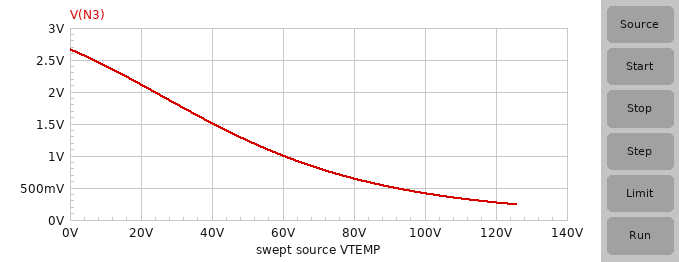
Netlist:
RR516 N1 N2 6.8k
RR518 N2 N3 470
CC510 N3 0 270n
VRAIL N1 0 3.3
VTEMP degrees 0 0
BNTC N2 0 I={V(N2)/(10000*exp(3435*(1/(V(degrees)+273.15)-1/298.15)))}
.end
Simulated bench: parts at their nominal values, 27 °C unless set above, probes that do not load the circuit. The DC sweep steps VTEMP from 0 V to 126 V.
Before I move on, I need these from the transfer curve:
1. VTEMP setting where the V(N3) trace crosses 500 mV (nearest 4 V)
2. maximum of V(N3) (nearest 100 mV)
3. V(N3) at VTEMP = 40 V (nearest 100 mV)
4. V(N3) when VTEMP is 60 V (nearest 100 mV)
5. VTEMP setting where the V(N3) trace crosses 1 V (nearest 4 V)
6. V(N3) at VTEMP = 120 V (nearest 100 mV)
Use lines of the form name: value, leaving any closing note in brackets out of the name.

VTEMP setting where the V(N3) trace crosses 500 mV: 92 V
maximum of V(N3): 2.7 V
V(N3) at VTEMP = 40 V: 1.5 V
V(N3) when VTEMP is 60 V: 1.0 V
VTEMP setting where the V(N3) trace crosses 1 V: 60 V
V(N3) at VTEMP = 120 V: 300 mV
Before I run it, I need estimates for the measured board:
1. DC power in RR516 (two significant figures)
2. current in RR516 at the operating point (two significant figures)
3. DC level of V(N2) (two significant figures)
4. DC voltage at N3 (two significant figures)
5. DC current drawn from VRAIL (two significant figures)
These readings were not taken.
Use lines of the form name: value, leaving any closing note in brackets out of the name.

DC power in RR516: 59 µW
current in RR516 at the operating point: 93 µA
DC level of V(N2): 2.7 V
DC voltage at N3: 2.7 V
DC current drawn from VRAIL: 93 µA
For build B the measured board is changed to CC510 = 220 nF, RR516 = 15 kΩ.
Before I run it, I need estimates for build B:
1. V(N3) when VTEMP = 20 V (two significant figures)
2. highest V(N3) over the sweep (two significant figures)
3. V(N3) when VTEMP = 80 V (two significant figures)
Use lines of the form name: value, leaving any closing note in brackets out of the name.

V(N3) when VTEMP = 20 V: 1.5 V
highest V(N3) over the sweep: 2.2 V
V(N3) when VTEMP = 80 V: 330 mV
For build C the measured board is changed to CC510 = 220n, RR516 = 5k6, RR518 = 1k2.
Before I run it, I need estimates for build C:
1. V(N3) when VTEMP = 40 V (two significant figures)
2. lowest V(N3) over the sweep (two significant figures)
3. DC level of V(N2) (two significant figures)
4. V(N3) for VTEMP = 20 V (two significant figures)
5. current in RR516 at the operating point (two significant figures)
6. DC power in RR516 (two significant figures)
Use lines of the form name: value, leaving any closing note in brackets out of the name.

V(N3) when VTEMP = 40 V: 1.7 V
lowest V(N3) over the sweep: 290 mV
DC level of V(N2): 2.8 V
V(N3) for VTEMP = 20 V: 2.3 V
current in RR516 at the operating point: 96 µA
DC power in RR516: 52 µW
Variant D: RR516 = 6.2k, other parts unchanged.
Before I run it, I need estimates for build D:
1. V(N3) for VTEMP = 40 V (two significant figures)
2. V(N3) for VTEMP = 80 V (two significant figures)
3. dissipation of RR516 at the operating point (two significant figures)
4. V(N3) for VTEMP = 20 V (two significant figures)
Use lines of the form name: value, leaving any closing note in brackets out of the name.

V(N3) for VTEMP = 40 V: 1.6 V
V(N3) for VTEMP = 80 V: 700 mV
dissipation of RR516 at the operating point: 55 µW
V(N3) for VTEMP = 20 V: 2.2 V
